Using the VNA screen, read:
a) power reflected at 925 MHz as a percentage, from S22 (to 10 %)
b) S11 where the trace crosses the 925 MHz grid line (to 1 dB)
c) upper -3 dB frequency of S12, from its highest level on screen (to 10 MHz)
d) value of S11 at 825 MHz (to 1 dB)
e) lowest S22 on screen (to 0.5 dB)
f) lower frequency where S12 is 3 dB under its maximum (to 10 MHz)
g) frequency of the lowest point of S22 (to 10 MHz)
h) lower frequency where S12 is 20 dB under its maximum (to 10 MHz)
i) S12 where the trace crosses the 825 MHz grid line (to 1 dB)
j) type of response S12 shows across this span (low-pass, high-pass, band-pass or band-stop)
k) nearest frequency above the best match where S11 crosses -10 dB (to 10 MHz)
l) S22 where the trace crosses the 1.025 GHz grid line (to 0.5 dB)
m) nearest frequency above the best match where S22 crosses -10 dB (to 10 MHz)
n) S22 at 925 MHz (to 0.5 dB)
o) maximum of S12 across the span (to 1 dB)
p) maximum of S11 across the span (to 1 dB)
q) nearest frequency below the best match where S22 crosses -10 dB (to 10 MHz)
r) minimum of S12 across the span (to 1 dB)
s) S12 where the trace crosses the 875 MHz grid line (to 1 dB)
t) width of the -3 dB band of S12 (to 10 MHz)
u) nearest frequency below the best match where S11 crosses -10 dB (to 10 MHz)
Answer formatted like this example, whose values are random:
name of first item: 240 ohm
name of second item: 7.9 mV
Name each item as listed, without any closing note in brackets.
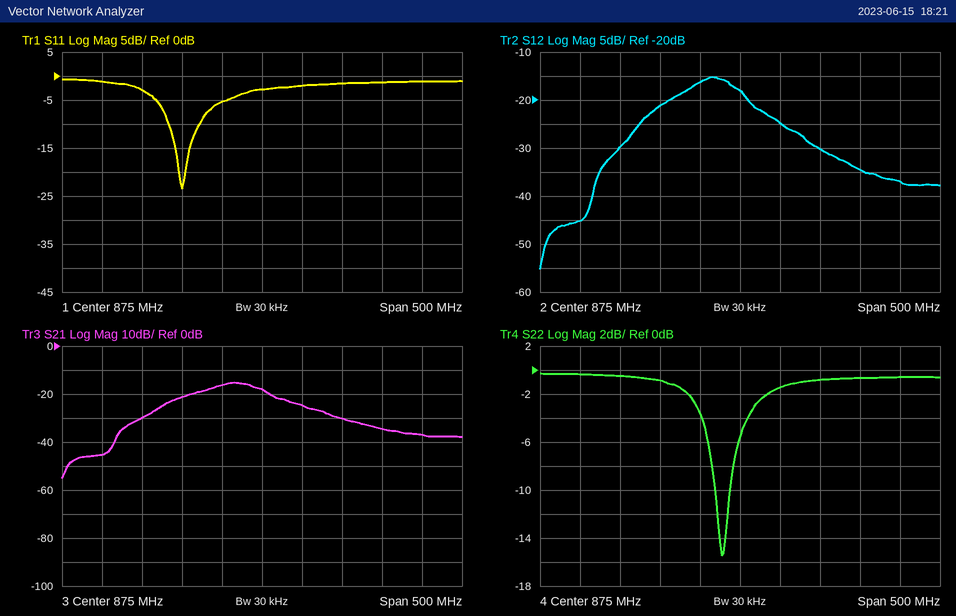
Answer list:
power reflected at 925 MHz as a percentage, from S22: 70 %
S11 where the trace crosses the 925 MHz grid line: -2 dB
upper -3 dB frequency of S12, from its highest level on screen: 880 MHz
value of S11 at 825 MHz: -5 dB
lowest S22 on screen: -15.5 dB
lower frequency where S12 is 3 dB under its maximum: 810 MHz
frequency of the lowest point of S22: 850 MHz
lower frequency where S12 is 20 dB under its maximum: 700 MHz
S12 where the trace crosses the 825 MHz grid line: -16 dB
type of response S12 shows across this span: band-pass
nearest frequency above the best match where S11 crosses -10 dB: 800 MHz
S22 where the trace crosses the 1.025 GHz grid line: -0.5 dB
nearest frequency above the best match where S22 crosses -10 dB: 860 MHz
S22 at 925 MHz: -1.5 dB
maximum of S12 across the span: -15 dB
maximum of S11 across the span: -1 dB
nearest frequency below the best match where S22 crosses -10 dB: 840 MHz
minimum of S12 across the span: -55 dB
S12 where the trace crosses the 875 MHz grid line: -18 dB
width of the -3 dB band of S12: 70 MHz
nearest frequency below the best match where S11 crosses -10 dB: 760 MHz
